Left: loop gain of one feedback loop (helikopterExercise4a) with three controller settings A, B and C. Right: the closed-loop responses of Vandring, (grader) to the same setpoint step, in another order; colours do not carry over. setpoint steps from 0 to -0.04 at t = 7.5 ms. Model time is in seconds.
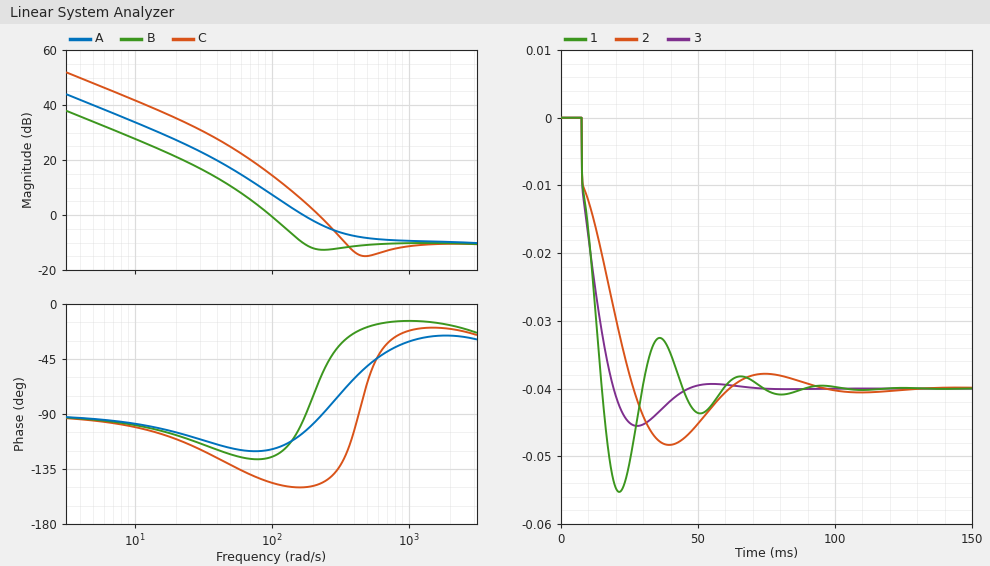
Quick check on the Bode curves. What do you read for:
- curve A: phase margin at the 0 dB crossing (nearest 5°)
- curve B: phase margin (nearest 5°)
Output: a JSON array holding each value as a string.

["75°", "55°"]
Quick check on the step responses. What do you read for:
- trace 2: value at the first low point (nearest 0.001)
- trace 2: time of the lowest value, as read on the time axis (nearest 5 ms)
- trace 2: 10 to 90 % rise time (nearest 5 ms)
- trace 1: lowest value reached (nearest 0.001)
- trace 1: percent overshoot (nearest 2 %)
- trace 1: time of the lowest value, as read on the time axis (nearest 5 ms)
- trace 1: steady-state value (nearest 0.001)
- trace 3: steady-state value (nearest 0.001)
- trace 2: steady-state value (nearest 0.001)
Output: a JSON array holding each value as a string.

["-0.048", "40 ms", "15 ms", "-0.055", "38 %", "20 ms", "-0.040", "-0.040", "-0.040"]
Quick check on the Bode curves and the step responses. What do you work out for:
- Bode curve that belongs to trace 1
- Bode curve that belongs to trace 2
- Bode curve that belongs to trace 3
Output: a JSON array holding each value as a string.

["C", "B", "A"]
